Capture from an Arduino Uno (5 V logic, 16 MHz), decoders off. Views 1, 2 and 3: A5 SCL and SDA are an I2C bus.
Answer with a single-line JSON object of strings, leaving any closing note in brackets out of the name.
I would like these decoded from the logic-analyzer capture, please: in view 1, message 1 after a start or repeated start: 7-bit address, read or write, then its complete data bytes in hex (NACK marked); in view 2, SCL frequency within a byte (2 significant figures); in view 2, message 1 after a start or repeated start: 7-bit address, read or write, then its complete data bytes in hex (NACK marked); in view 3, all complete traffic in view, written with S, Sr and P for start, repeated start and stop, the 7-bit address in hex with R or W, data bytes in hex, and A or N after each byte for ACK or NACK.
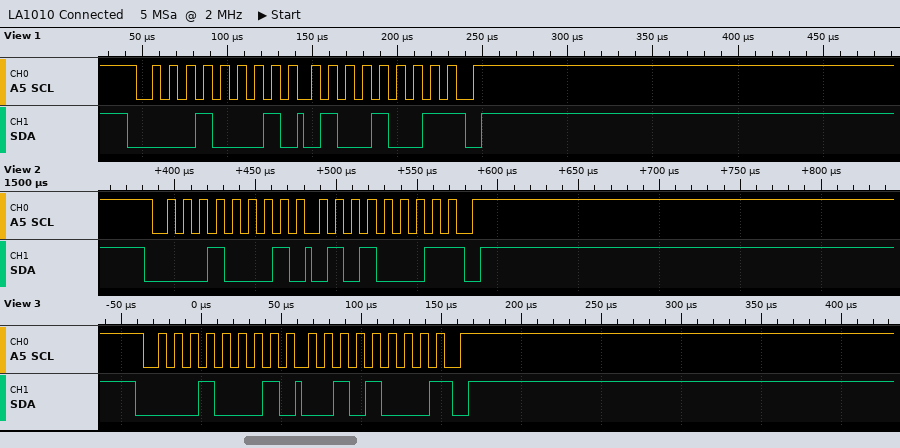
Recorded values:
{"in view 1, message 1 after a start or repeated start: 7-bit address, read or write, then its complete data bytes in hex": "0x08 read: 49 NACK", "in view 2, SCL frequency within a byte": "100 kHz", "in view 2, message 1 after a start or repeated start: 7-bit address, read or write, then its complete data bytes in hex": "0x08 read: 51 NACK", "in view 3, all complete traffic in view, written with S, Sr and P for start, repeated start and stop, the 7-bit address in hex with R or W, data bytes in hex, and A or N after each byte for ACK or NACK": "S 08R A 28 N P"}
